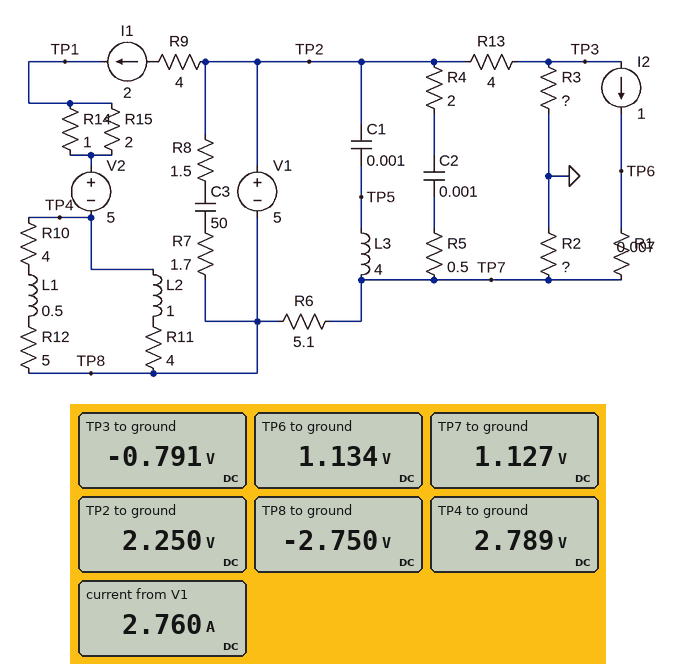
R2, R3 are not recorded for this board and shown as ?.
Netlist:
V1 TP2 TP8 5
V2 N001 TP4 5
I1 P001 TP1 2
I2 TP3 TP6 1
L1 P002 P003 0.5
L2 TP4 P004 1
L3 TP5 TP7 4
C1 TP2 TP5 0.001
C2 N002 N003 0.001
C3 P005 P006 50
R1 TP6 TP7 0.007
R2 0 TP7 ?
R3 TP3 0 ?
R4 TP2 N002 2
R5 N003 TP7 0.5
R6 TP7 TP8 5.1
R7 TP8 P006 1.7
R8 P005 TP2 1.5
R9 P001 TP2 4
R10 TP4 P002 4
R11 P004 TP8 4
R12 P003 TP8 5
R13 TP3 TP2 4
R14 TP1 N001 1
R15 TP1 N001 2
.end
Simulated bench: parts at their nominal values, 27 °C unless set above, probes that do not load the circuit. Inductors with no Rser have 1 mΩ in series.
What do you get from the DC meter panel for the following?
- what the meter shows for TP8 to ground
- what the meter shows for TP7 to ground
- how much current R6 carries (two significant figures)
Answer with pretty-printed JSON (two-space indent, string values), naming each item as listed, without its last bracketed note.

{
  "what the meter shows for TP8 to ground": "-2.750 V",
  "what the meter shows for TP7 to ground": "1.127 V",
  "how much current R6 carries": "760 mA"
}
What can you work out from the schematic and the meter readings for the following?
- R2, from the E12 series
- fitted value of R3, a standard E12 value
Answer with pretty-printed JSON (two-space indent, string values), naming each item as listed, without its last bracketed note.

{
  "R2, from the E12 series": "4.7 Ω",
  "fitted value of R3, a standard E12 value": "3.3 Ω"
}
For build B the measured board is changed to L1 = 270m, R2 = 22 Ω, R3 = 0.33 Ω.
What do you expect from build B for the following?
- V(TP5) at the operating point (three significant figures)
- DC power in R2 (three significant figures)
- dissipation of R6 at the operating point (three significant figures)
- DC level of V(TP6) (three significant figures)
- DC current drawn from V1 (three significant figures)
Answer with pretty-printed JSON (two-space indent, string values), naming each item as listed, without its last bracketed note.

{
  "V(TP5) at the operating point": "2.87 V",
  "DC power in R2": "374 mW",
  "dissipation of R6 at the operating point": "3.86 W",
  "DC level of V(TP6)": "2.88 V",
  "DC current drawn from V1": "2.87 A"
}
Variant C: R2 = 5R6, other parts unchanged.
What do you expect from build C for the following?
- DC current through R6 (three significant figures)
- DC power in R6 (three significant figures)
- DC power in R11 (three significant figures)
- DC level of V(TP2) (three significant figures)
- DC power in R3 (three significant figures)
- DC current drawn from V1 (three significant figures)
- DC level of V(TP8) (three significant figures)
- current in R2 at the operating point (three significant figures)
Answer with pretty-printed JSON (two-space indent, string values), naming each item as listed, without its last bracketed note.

{
  "DC current through R6": "772 mA",
  "DC power in R6": "3.04 W",
  "DC power in R11": "7.67 W",
  "DC level of V(TP2)": "2.34 V",
  "DC power in R3": "171 mW",
  "DC current drawn from V1": "2.77 A",
  "DC level of V(TP8)": "-2.66 V",
  "current in R2 at the operating point": "228 mA"
}
